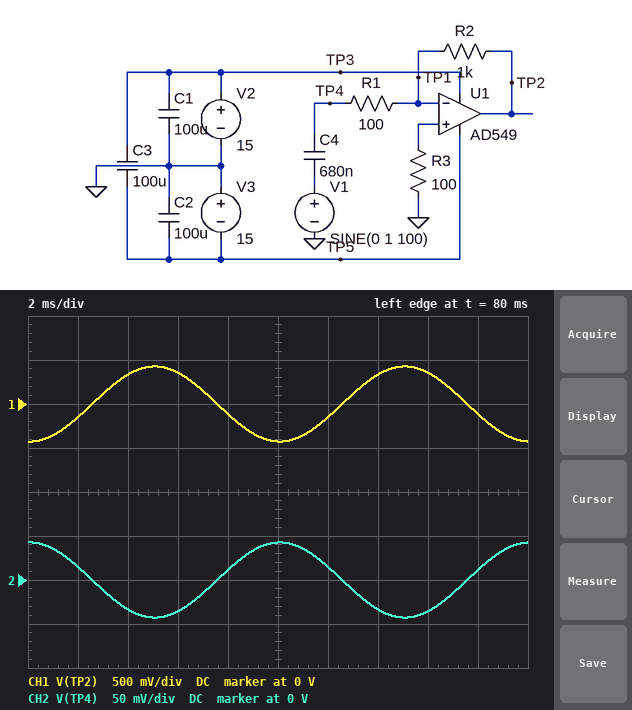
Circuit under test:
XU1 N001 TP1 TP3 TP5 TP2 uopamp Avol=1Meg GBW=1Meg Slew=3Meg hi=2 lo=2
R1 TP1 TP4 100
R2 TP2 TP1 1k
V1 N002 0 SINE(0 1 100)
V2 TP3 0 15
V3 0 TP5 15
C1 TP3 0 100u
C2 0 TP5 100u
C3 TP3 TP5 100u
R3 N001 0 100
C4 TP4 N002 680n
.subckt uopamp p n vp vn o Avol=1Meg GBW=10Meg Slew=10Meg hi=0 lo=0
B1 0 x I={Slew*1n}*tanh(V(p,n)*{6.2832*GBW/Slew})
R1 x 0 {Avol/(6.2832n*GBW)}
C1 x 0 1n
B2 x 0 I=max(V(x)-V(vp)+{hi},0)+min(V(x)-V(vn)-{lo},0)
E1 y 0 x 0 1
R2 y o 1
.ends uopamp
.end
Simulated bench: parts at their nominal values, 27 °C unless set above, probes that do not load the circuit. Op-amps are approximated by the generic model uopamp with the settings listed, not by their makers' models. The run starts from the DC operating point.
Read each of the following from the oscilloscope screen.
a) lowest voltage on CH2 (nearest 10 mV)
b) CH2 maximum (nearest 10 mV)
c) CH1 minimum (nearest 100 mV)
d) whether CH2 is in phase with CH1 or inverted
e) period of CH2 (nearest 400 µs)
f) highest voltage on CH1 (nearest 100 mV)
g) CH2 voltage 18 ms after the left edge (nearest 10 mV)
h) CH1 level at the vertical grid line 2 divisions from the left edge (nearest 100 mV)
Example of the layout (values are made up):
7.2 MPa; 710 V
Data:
-40 mV; 40 mV; -400 mV; inverted; 10.0 ms; 400 mV; 10 mV; 300 mV
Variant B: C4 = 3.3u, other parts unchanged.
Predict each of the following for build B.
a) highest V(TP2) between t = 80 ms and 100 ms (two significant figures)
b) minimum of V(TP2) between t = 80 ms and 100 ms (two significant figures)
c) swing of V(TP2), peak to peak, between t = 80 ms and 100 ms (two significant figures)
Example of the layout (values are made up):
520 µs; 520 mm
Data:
2.0 V; -2.0 V; 4.1 V
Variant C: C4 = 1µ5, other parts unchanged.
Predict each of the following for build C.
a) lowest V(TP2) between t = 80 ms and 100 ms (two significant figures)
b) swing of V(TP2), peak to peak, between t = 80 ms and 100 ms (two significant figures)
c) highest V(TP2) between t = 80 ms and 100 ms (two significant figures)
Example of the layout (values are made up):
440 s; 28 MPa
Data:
-940 mV; 1.9 V; 940 mV
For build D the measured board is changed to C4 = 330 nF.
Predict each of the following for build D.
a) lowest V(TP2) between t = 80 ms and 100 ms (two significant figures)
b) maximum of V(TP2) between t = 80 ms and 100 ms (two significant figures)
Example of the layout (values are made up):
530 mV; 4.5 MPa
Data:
-210 mV; 210 mV
